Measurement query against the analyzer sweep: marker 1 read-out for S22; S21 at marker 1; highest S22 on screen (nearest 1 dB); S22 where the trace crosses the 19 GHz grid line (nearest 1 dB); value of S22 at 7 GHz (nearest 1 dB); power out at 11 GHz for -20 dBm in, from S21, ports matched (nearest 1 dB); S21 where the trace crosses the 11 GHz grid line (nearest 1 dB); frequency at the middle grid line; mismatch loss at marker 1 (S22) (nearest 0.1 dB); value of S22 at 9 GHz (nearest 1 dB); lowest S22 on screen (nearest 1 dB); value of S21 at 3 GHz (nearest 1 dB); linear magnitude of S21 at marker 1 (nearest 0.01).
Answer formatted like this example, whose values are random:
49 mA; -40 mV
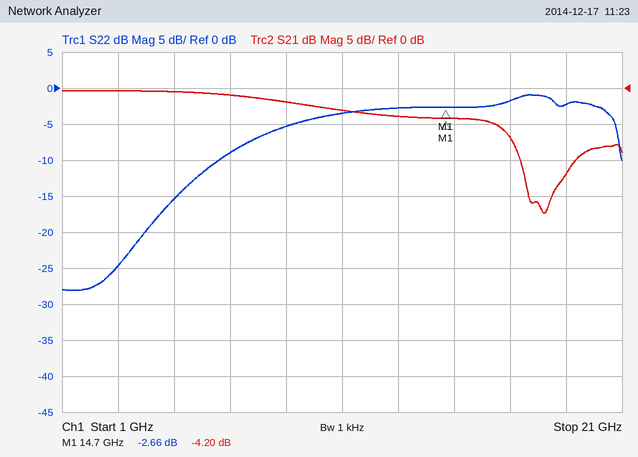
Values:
-2.66 dB; -4.20 dB; -1 dB; -2 dB; -9 dB; -23 dBm; -3 dB; 11 GHz; 3.4 dB; -5 dB; -28 dB; 0 dB; 0.62
